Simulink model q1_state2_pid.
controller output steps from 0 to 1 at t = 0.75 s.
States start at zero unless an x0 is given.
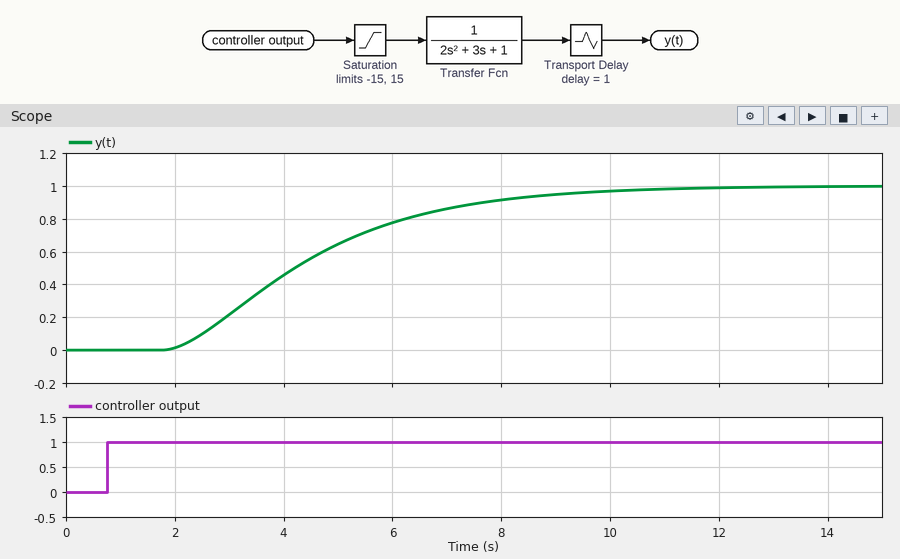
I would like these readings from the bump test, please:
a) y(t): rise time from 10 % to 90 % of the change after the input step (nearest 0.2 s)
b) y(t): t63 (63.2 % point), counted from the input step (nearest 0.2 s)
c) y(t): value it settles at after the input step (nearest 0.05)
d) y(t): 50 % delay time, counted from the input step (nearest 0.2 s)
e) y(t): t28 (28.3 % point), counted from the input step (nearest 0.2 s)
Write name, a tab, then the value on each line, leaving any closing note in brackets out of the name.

y(t): rise time from 10 % to 90 % of the change after the input step	5.2 s
y(t): t63 (63.2 % point), counted from the input step	4.2 s
y(t): value it settles at after the input step	1.00
y(t): 50 % delay time, counted from the input step	3.4 s
y(t): t28 (28.3 % point), counted from the input step	2.6 s
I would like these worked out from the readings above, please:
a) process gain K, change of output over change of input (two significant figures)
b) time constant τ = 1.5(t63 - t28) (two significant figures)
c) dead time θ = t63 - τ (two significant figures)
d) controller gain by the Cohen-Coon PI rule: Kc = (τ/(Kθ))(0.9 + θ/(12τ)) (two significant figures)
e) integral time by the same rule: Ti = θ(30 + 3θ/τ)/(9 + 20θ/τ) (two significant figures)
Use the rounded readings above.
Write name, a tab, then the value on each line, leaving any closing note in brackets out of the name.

process gain K, change of output over change of input	1.0
time constant τ = 1.5(t63 - t28)	2.4 s
dead time θ = t63 - τ	1.8 s
controller gain by the Cohen-Coon PI rule: Kc = (τ/(Kθ))(0.9 + θ/(12τ))	1.3
integral time by the same rule: Ti = θ(30 + 3θ/τ)/(9 + 20θ/τ)	2.4 s
